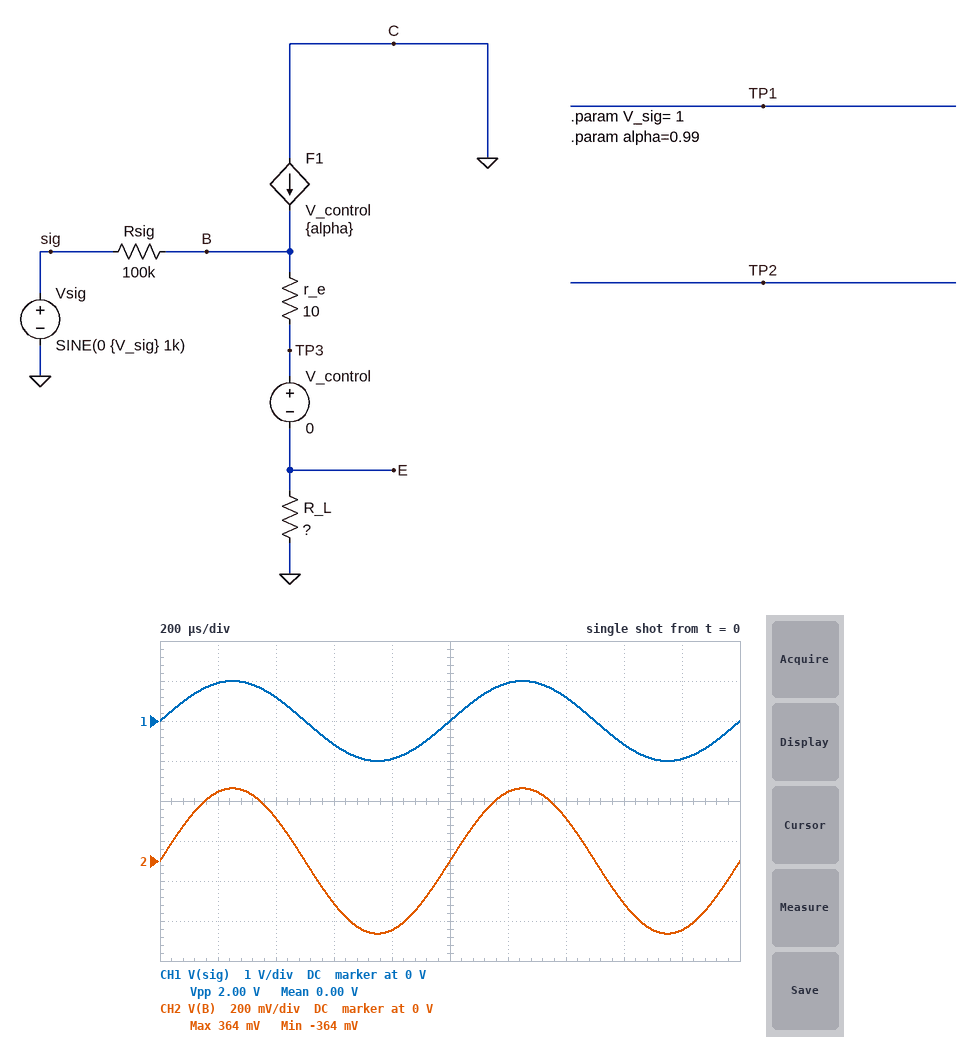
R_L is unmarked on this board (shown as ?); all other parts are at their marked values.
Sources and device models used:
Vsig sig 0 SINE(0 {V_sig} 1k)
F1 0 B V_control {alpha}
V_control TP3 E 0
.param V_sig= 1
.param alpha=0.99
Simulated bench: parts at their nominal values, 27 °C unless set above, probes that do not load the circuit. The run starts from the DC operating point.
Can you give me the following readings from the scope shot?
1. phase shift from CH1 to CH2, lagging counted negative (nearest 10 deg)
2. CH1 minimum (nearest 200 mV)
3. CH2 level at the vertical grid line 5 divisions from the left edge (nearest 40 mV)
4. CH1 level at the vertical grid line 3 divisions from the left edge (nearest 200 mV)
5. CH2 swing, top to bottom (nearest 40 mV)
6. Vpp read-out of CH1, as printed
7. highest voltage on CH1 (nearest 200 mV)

0 deg
-1.0 V
0 V
-600 mV
720 mV
2.00 V
1.0 V
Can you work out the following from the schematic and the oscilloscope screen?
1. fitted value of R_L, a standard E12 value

560 Ω
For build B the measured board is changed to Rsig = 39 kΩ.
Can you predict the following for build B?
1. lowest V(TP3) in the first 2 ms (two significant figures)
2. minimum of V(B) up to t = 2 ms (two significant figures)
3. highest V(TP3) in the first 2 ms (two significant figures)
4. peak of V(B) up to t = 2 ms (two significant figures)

-580 mV
-590 mV
580 mV
590 mV
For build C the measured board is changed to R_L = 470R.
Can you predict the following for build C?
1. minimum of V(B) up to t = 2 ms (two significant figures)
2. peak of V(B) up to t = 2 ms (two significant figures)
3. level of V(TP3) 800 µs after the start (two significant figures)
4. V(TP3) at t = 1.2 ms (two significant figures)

-320 mV
320 mV
-300 mV
300 mV
